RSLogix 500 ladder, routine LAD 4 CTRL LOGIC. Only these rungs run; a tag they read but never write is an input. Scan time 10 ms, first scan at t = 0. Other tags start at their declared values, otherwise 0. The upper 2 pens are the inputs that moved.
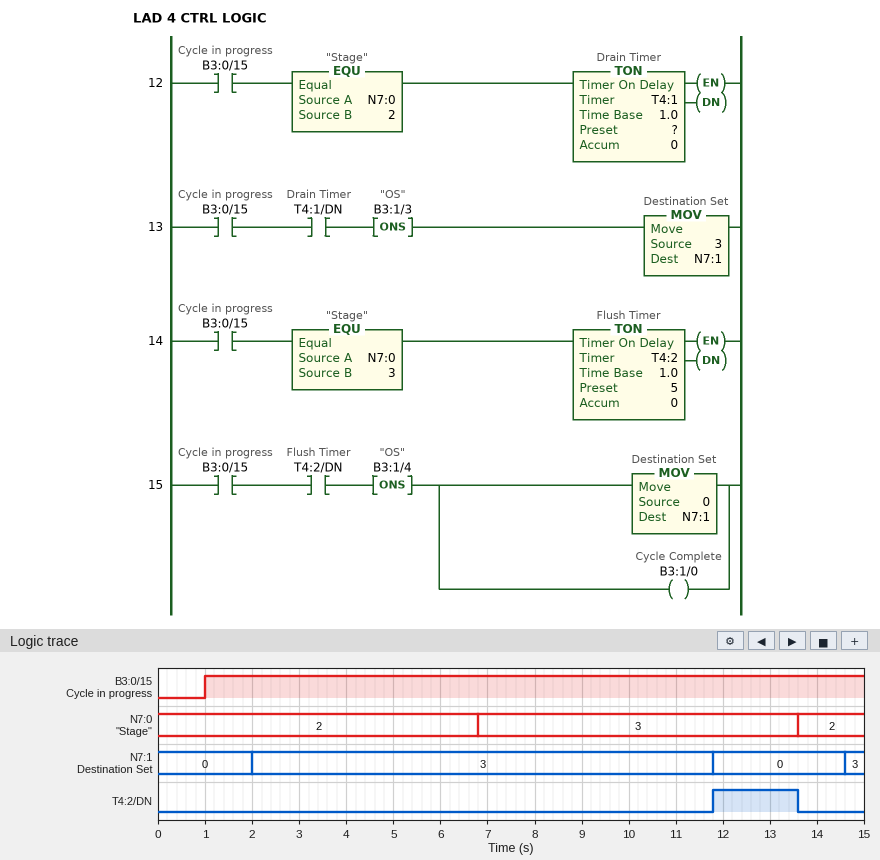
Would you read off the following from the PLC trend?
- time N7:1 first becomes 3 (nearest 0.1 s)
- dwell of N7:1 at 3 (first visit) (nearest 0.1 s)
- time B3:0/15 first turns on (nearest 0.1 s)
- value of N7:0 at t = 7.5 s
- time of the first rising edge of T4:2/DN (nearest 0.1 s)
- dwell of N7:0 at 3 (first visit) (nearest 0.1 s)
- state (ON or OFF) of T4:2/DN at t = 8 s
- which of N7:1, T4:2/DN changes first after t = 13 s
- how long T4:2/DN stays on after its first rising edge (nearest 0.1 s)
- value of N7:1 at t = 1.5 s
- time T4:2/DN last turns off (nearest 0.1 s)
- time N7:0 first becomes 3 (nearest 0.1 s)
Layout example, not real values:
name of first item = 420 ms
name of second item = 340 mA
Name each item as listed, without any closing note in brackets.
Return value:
time N7:1 first becomes 3 = 2.0 s
dwell of N7:1 at 3 (first visit) = 9.8 s
time B3:0/15 first turns on = 1.0 s
value of N7:0 at t = 7.5 s = 3
time of the first rising edge of T4:2/DN = 11.8 s
dwell of N7:0 at 3 (first visit) = 6.8 s
state (ON or OFF) of T4:2/DN at t = 8 s = OFF
which of N7:1, T4:2/DN changes first after t = 13 s = T4:2/DN
how long T4:2/DN stays on after its first rising edge = 1.8 s
value of N7:1 at t = 1.5 s = 0
time T4:2/DN last turns off = 13.6 s
time N7:0 first becomes 3 = 6.8 s
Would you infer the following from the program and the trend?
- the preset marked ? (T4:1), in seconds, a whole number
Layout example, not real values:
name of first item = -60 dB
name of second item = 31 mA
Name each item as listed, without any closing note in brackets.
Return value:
the preset marked ? (T4:1), in seconds, a whole number = 1 s
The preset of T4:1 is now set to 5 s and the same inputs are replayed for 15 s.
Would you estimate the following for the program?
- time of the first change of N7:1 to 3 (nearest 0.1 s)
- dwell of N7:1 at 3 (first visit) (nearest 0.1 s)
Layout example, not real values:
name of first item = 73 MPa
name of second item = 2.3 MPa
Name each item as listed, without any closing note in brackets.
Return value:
time of the first change of N7:1 to 3 = 6.0 s
dwell of N7:1 at 3 (first visit) = 5.8 s
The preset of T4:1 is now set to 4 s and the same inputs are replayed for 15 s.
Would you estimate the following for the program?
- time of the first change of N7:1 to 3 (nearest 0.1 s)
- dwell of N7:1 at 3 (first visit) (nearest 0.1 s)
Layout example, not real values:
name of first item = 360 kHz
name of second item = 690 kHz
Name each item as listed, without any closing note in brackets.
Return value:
time of the first change of N7:1 to 3 = 5.0 s
dwell of N7:1 at 3 (first visit) = 6.8 s
